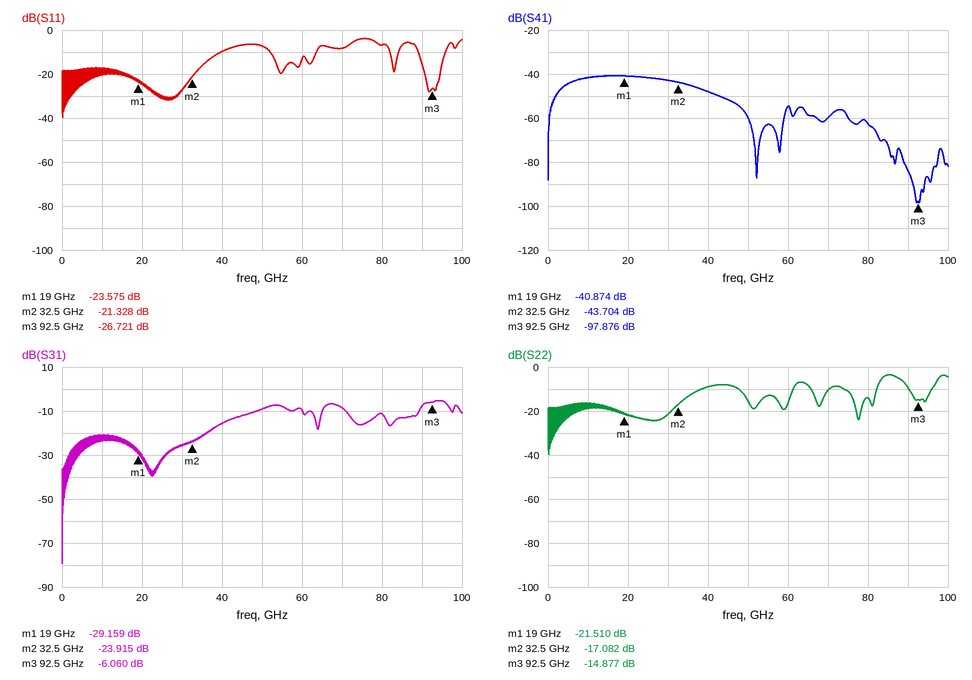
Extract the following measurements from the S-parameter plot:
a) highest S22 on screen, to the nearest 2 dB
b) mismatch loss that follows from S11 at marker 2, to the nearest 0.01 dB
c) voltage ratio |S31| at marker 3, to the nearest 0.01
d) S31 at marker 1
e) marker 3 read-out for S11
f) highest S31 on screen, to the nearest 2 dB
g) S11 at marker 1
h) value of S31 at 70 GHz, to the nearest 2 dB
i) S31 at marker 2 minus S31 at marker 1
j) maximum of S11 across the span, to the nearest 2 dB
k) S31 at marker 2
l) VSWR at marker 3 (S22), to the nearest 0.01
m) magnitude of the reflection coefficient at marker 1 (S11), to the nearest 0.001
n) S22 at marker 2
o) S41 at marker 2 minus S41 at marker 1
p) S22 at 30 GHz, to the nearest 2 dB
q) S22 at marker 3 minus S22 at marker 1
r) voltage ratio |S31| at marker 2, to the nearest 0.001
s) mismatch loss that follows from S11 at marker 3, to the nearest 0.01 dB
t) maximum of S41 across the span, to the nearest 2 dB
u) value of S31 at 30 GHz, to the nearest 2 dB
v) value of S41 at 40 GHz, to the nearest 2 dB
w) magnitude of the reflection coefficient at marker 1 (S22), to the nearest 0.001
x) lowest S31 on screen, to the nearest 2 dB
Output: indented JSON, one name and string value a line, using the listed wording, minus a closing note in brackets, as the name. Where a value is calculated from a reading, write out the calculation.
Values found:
{
  "highest S22 on screen, to the nearest 2 dB": "-4 dB",
  "mismatch loss that follows from S11 at marker 2, to the nearest 0.01 dB": "−10 log10(1 − 10^(-21.328/10)) ≈ 0.03 dB",
  "voltage ratio |S31| at marker 3, to the nearest 0.01": "10^(-6.06/20) ≈ 0.50",
  "S31 at marker 1": "-29.159 dB",
  "marker 3 read-out for S11": "-26.721 dB",
  "highest S31 on screen, to the nearest 2 dB": "-6 dB",
  "S11 at marker 1": "-23.575 dB",
  "value of S31 at 70 GHz, to the nearest 2 dB": "-8 dB",
  "S31 at marker 2 minus S31 at marker 1": "-23.915 − (-29.159) = 5.244 dB",
  "maximum of S11 across the span, to the nearest 2 dB": "-4 dB",
  "S31 at marker 2": "-23.915 dB",
  "VSWR at marker 3 (S22), to the nearest 0.01": "(1 + 0.1804)/(1 − 0.1804) ≈ 1.44",
  "magnitude of the reflection coefficient at marker 1 (S11), to the nearest 0.001": "10^(-23.575/20) ≈ 0.066",
  "S22 at marker 2": "-17.082 dB",
  "S41 at marker 2 minus S41 at marker 1": "-43.704 − (-40.874) = -2.830 dB",
  "S22 at 30 GHz, to the nearest 2 dB": "-22 dB",
  "S22 at marker 3 minus S22 at marker 1": "-14.877 − (-21.51) = 6.633 dB",
  "voltage ratio |S31| at marker 2, to the nearest 0.001": "10^(-23.915/20) ≈ 0.064",
  "mismatch loss that follows from S11 at marker 3, to the nearest 0.01 dB": "−10 log10(1 − 10^(-26.721/10)) ≈ 0.01 dB",
  "maximum of S41 across the span, to the nearest 2 dB": "-40 dB",
  "value of S31 at 30 GHz, to the nearest 2 dB": "-26 dB",
  "value of S41 at 40 GHz, to the nearest 2 dB": "-48 dB",
  "magnitude of the reflection coefficient at marker 1 (S22), to the nearest 0.001": "10^(-21.51/20) ≈ 0.084",
  "lowest S31 on screen, to the nearest 2 dB": "-80 dB"
}
